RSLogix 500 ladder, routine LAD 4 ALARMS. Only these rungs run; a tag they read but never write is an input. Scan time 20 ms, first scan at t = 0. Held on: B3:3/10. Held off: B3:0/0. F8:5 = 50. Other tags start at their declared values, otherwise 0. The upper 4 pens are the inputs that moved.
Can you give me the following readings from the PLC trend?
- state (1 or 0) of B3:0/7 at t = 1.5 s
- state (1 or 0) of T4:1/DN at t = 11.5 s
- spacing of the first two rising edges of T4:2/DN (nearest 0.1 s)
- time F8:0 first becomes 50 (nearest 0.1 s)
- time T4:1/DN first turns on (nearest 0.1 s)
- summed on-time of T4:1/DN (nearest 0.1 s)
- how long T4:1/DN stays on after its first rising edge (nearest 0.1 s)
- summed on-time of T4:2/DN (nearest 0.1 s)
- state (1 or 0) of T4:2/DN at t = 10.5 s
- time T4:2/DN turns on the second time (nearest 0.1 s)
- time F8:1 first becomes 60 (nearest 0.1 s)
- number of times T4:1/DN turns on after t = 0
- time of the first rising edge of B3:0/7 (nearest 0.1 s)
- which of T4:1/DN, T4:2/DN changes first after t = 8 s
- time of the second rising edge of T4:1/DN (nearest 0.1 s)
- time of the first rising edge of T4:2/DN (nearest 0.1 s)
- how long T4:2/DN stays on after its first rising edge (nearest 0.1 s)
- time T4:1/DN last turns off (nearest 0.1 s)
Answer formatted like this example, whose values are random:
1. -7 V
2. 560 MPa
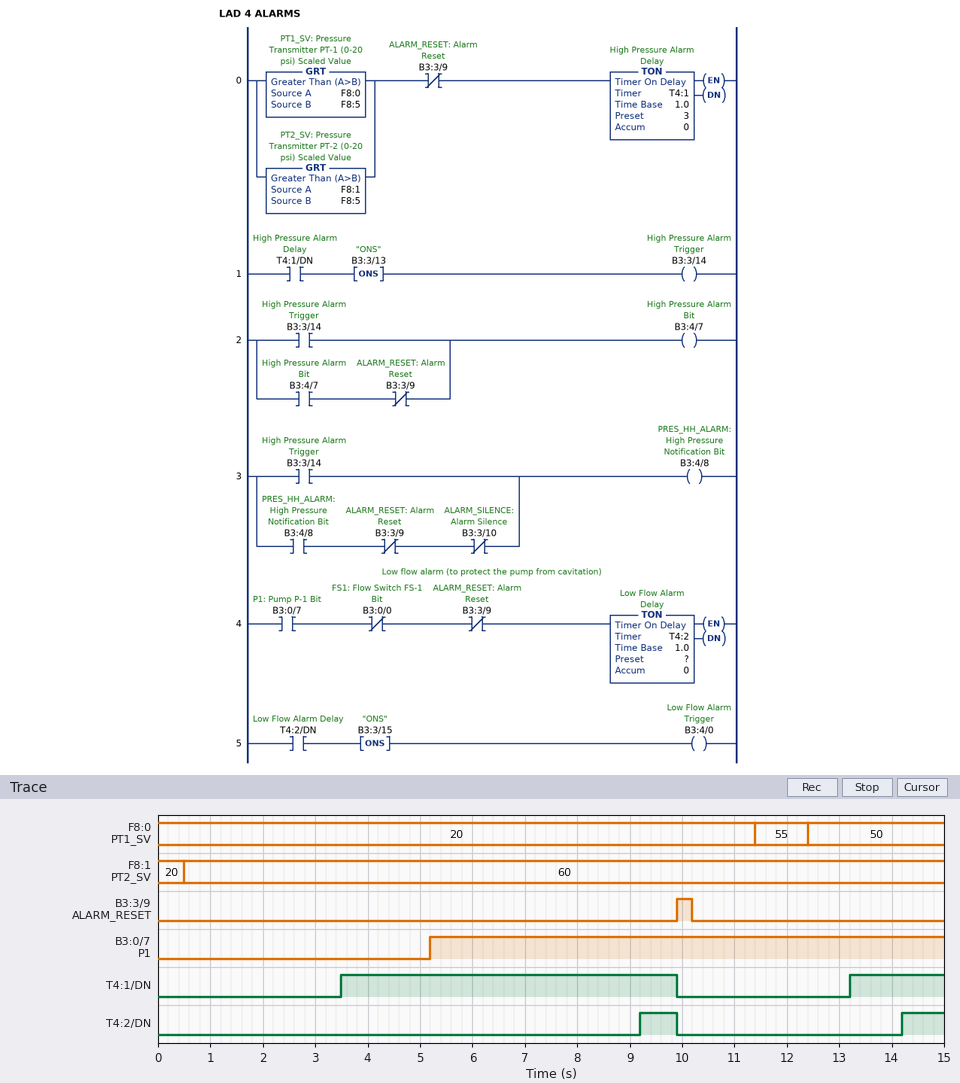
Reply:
1. 0
2. 0
3. 5.0 s
4. 12.4 s
5. 3.5 s
6. 8.2 s
7. 6.4 s
8. 1.5 s
9. 0
10. 14.2 s
11. 0.5 s
12. 2
13. 5.2 s
14. T4:2/DN
15. 13.2 s
16. 9.2 s
17. 0.7 s
18. 9.9 s
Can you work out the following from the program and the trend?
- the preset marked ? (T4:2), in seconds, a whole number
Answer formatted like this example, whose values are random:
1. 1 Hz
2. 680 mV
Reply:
1. 4 s
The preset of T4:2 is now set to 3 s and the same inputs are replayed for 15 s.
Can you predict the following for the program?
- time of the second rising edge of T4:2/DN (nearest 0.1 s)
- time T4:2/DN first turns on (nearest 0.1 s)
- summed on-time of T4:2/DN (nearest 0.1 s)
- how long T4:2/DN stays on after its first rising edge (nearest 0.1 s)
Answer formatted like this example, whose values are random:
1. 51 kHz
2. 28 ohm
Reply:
1. 13.2 s
2. 8.2 s
3. 3.5 s
4. 1.7 s
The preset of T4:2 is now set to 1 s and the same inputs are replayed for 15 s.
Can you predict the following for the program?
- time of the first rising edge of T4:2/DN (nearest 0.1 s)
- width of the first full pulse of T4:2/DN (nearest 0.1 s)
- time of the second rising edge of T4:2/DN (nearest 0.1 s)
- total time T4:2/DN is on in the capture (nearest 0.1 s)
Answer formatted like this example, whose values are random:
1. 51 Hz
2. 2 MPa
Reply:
1. 6.2 s
2. 3.7 s
3. 11.2 s
4. 7.5 s
